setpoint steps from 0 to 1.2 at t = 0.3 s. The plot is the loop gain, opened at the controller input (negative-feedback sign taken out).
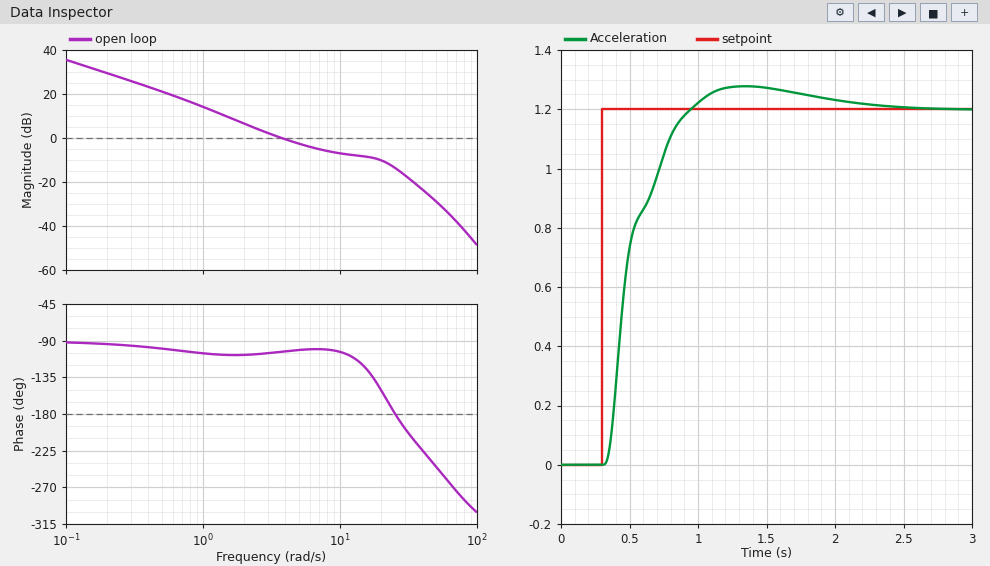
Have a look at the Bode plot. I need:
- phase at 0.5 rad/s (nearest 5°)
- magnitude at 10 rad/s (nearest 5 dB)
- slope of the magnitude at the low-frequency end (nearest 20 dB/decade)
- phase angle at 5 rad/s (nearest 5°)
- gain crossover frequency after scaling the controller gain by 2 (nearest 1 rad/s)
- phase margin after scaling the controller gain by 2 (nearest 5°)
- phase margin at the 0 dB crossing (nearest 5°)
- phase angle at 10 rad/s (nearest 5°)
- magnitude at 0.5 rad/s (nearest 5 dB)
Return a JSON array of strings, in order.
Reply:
["-100°", "-5 dB", "-20 dB/decade", "-100°", "8 rad/s", "80°", "75°", "-105°", "20 dB"]
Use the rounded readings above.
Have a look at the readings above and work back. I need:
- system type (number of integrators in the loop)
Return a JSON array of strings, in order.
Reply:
["1"]
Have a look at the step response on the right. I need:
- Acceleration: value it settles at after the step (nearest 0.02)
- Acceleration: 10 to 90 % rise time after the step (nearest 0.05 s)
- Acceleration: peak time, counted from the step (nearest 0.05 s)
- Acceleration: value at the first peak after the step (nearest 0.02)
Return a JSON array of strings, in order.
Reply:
["1.20", "0.40 s", "1.05 s", "1.28"]
